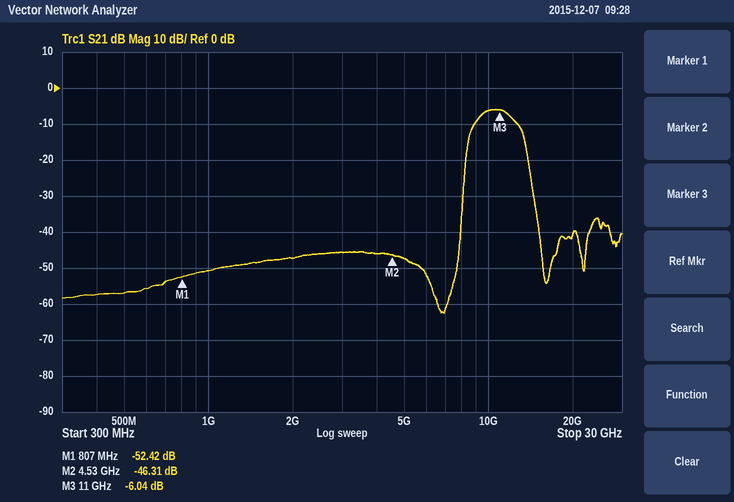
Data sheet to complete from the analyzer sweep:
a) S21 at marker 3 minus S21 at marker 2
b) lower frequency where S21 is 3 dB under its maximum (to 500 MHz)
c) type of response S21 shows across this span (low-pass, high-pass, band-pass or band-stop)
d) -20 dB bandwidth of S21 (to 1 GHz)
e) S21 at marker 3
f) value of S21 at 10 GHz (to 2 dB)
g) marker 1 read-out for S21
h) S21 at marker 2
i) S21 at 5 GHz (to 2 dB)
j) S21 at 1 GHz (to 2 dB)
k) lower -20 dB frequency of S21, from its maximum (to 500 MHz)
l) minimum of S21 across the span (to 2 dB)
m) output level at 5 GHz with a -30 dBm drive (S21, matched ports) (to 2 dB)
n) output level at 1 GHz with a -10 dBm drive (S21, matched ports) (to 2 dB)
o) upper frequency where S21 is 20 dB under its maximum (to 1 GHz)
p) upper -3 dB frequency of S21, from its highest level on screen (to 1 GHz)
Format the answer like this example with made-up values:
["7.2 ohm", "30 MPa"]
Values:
["40.27 dB", "9.0 GHz", "band-pass", "6 GHz", "-6.04 dB", "-6 dB", "-52.42 dB", "-46.31 dB", "-48 dB", "-50 dB", "8.0 GHz", "-62 dB", "-78 dBm", "-60 dBm", "14 GHz", "12 GHz"]
